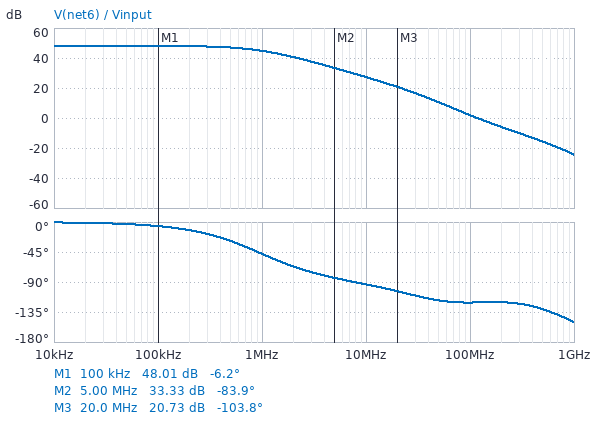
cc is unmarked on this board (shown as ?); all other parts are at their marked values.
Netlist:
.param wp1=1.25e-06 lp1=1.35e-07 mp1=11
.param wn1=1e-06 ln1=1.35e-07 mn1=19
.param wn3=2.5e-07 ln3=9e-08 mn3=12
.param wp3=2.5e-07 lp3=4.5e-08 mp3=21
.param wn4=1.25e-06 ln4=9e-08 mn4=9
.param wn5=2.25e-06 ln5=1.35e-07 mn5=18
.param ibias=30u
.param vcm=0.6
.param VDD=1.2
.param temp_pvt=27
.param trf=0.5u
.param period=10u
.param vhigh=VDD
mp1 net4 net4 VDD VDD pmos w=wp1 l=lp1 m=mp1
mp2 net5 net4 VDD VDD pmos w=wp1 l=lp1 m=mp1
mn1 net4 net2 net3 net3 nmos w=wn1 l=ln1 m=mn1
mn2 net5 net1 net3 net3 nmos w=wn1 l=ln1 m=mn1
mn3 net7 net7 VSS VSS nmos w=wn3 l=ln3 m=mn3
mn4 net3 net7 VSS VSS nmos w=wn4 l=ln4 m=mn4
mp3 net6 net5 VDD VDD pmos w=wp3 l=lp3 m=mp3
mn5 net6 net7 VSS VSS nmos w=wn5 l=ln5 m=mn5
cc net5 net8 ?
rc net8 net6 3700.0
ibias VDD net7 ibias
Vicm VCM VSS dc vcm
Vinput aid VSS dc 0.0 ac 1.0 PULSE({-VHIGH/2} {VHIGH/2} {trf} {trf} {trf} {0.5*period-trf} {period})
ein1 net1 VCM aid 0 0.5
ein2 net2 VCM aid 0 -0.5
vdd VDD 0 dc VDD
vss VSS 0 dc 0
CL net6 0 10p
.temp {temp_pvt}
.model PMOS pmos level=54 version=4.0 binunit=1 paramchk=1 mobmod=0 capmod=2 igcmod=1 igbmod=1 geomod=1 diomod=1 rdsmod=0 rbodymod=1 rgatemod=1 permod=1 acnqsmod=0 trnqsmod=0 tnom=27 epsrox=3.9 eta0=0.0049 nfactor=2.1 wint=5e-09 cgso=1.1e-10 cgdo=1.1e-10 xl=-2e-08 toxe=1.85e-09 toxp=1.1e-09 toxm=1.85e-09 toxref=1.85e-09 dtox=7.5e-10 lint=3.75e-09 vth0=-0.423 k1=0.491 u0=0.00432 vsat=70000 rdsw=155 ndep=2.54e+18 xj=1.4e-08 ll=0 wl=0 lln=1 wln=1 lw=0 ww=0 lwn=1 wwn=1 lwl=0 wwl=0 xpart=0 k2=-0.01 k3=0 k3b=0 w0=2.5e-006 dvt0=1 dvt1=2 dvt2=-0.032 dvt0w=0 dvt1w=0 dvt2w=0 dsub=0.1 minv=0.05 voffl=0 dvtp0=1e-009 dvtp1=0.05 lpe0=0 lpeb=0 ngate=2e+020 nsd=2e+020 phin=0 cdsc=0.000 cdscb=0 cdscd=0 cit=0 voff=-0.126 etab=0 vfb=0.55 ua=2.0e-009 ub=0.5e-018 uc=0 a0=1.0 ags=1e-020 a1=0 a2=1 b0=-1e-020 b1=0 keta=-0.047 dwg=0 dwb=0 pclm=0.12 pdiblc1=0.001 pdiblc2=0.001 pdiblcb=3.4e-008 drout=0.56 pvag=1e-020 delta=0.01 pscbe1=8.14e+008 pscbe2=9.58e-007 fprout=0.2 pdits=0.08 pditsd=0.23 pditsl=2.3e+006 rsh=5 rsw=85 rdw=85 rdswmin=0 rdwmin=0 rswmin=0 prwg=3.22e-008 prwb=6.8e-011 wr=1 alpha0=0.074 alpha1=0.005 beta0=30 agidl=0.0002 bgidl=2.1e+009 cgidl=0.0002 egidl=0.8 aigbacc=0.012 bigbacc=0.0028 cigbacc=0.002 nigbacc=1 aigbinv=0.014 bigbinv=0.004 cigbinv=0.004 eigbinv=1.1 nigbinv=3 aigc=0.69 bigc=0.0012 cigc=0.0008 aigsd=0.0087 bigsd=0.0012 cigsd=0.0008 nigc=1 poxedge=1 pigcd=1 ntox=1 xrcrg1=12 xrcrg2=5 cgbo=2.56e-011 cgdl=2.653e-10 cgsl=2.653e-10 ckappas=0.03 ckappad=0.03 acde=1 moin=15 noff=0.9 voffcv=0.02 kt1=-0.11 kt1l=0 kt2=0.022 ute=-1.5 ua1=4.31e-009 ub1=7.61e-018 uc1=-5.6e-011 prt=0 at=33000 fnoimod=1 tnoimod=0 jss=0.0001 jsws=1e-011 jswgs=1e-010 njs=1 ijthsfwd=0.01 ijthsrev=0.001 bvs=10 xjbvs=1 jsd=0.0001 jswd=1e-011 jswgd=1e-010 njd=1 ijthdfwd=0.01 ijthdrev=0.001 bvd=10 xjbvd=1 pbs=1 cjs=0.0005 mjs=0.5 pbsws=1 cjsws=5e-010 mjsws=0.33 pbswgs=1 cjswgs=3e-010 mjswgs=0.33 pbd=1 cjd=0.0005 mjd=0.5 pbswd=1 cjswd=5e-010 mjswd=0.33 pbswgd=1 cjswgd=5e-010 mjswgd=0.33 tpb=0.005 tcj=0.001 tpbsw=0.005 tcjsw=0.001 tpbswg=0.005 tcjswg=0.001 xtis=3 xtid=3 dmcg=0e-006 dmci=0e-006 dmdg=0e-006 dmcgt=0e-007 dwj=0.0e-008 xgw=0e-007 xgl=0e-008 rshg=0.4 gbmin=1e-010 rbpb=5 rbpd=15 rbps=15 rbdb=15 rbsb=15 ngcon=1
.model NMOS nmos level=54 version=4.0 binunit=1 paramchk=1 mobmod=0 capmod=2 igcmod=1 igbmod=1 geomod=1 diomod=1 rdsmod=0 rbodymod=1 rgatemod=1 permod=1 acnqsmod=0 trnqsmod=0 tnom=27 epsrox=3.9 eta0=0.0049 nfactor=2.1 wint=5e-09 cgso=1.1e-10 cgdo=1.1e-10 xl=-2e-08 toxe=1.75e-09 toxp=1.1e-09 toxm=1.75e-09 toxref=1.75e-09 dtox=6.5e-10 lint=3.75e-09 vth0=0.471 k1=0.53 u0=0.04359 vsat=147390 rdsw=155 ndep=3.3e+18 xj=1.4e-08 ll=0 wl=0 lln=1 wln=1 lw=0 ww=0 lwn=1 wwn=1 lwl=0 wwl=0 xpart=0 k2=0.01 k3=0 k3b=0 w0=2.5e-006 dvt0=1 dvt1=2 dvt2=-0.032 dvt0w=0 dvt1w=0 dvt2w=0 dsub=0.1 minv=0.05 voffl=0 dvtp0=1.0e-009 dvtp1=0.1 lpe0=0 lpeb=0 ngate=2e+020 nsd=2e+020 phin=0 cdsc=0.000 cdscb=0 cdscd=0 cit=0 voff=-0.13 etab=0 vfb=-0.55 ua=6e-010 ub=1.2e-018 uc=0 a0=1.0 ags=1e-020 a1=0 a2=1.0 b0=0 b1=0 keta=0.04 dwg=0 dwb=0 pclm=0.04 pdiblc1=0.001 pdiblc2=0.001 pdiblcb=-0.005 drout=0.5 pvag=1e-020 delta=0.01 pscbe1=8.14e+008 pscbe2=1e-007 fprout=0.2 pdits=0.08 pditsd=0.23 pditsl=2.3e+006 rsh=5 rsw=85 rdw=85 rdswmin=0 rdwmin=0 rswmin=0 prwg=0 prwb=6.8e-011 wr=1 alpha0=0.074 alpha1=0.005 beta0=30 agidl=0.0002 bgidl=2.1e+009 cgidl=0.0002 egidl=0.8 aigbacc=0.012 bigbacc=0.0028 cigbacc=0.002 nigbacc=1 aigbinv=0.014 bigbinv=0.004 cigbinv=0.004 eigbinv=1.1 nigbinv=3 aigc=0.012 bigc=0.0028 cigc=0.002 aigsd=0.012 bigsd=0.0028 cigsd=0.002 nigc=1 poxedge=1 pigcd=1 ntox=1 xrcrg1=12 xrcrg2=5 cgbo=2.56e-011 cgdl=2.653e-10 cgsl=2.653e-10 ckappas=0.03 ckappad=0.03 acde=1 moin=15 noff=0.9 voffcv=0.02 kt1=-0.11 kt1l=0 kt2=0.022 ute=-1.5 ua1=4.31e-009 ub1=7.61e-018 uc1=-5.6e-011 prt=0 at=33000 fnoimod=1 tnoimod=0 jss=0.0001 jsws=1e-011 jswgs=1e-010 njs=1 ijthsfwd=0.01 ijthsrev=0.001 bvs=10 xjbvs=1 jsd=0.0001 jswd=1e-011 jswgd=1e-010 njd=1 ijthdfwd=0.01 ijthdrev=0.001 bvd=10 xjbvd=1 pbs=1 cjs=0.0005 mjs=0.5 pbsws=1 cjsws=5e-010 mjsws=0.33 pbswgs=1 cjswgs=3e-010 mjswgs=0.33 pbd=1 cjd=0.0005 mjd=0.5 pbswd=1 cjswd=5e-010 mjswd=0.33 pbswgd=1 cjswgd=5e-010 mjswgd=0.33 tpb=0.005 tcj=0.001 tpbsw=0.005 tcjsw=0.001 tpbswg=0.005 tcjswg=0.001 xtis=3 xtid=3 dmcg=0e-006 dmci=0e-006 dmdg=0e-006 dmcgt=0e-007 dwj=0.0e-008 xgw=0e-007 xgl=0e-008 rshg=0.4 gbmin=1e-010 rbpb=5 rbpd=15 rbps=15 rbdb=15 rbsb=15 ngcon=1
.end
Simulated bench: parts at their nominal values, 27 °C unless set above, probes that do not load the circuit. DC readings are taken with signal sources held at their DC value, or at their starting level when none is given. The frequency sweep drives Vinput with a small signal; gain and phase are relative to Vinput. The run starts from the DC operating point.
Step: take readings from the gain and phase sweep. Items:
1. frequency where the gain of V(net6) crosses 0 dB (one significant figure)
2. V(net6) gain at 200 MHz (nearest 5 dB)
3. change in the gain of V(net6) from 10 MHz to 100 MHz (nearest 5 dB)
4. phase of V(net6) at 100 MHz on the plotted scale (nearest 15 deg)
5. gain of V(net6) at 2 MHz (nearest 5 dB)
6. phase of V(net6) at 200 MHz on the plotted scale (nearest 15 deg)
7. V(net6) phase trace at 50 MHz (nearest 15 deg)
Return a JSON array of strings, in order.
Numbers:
["100 MHz", "-5 dB", "-25 dB", "-120 deg", "40 dB", "-120 deg", "-120 deg"]
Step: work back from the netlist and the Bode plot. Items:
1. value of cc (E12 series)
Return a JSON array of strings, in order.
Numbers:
["470 fF"]
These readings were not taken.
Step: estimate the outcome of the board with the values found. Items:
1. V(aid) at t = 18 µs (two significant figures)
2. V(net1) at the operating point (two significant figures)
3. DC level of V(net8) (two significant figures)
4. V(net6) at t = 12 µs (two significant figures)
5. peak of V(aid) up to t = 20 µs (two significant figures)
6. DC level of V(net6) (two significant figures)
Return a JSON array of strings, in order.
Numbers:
["-600 mV", "600 mV", "870 mV", "1.2 V", "600 mV", "870 mV"]
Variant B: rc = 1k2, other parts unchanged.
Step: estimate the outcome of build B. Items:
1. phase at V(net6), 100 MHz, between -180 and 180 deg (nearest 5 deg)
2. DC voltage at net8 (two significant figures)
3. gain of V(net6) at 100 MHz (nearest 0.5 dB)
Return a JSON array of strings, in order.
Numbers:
["-150 deg", "870 mV", "-0.5 dB"]
